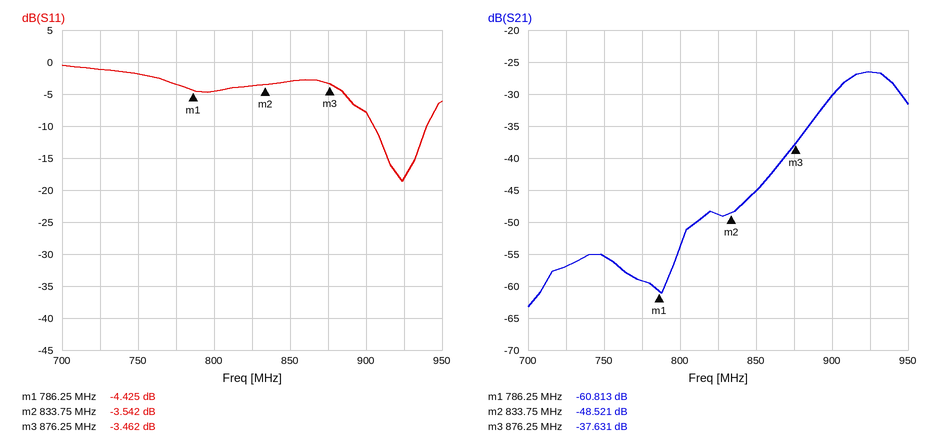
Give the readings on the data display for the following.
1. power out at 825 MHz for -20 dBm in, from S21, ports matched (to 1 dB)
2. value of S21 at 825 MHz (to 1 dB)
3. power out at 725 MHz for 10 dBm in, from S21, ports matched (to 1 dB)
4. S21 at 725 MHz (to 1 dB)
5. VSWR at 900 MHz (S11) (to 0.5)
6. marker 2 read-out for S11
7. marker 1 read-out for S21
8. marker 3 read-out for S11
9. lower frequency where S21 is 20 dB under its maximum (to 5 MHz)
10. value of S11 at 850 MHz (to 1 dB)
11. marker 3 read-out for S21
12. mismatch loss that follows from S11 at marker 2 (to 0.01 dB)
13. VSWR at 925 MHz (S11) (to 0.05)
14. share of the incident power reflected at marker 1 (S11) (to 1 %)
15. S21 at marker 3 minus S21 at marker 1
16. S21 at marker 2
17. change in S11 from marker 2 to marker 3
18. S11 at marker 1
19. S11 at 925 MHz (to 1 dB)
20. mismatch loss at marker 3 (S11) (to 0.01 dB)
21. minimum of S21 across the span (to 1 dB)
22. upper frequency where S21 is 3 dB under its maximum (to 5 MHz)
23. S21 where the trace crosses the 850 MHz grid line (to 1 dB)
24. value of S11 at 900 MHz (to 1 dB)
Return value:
-69 dBm
-49 dB
-47 dBm
-57 dB
2.5
-3.542 dB
-60.813 dB
-3.462 dB
845 MHz
-3 dB
-37.631 dB
2.54 dB
1.30
36 %
23.182 dB
-48.521 dB
0.080 dB
-4.425 dB
-18 dB
2.60 dB
-63 dB
945 MHz
-45 dB
-8 dB
